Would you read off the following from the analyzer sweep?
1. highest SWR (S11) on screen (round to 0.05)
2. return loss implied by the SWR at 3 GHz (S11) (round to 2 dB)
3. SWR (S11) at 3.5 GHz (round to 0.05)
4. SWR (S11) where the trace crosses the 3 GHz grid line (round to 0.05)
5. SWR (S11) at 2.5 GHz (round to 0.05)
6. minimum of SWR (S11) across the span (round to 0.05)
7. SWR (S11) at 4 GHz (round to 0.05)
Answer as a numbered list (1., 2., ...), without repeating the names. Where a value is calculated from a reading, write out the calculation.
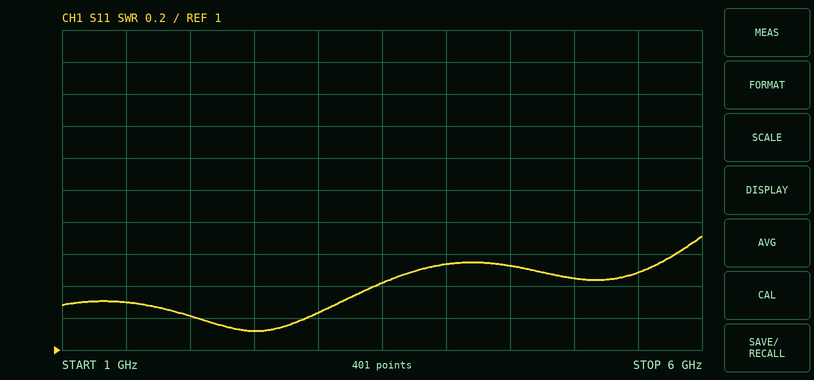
1. 1.70
2. −20 log10((1.25 − 1)/(1.25 + 1)) ≈ 19.1 dB, so 20 dB to the nearest 2 dB
3. 1.40
4. 1.25
5. 1.10
6. 1.10
7. 1.55
